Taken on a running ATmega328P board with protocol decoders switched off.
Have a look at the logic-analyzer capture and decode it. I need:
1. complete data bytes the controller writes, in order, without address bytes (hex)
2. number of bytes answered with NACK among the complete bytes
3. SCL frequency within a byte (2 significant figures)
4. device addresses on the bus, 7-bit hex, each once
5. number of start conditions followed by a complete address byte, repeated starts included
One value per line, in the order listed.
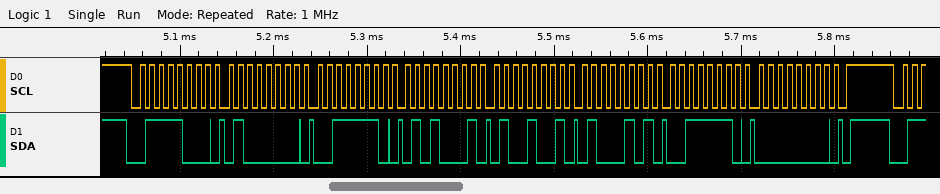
40 3E 51 49 45 3E 00
0
100 kHz
0x3C
1
